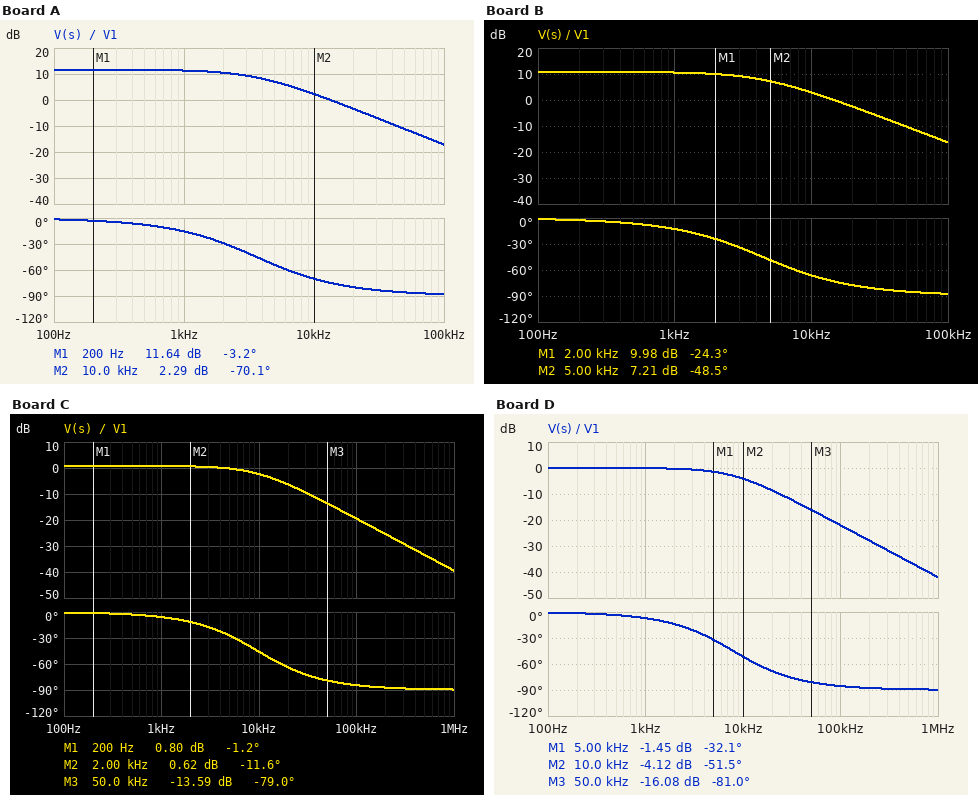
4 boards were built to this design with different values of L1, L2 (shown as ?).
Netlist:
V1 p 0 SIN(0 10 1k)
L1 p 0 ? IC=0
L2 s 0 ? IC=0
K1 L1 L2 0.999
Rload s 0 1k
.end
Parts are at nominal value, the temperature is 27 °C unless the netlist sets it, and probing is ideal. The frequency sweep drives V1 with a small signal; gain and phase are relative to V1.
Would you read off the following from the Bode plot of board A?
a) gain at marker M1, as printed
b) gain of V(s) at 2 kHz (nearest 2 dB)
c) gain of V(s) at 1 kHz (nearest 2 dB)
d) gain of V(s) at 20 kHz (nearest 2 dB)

11.64 dB
10 dB
12 dB
-4 dB
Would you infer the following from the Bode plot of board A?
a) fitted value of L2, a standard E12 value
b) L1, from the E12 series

22 H
1.5 H
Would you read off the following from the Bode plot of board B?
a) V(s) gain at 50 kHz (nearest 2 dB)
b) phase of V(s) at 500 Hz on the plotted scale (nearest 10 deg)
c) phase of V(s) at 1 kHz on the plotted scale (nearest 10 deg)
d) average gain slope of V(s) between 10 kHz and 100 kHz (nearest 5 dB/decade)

-10 dB
-10 deg
-10 deg
-20 dB/decade
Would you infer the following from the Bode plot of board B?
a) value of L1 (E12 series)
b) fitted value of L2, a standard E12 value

1.5 H
18 H
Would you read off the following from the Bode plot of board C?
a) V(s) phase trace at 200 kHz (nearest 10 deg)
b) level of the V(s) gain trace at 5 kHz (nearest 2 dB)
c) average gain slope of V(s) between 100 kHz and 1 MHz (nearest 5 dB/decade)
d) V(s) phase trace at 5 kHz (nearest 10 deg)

-90 deg
0 dB
-20 dB/decade
-30 deg
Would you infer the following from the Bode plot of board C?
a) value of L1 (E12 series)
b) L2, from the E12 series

6.8 H
8.2 H
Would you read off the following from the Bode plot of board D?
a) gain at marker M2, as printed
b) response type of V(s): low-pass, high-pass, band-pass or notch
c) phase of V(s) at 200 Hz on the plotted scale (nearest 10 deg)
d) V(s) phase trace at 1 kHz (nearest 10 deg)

-4.12 dB
low-pass
0 deg
-10 deg
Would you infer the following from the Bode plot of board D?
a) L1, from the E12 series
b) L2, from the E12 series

10 H
10 H
